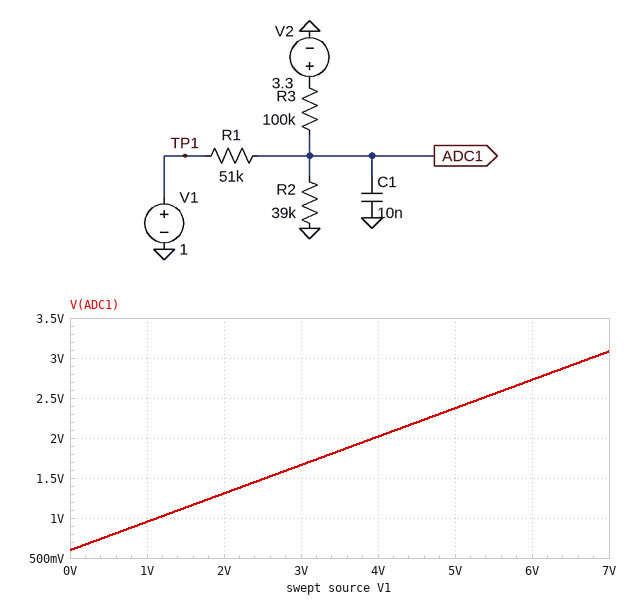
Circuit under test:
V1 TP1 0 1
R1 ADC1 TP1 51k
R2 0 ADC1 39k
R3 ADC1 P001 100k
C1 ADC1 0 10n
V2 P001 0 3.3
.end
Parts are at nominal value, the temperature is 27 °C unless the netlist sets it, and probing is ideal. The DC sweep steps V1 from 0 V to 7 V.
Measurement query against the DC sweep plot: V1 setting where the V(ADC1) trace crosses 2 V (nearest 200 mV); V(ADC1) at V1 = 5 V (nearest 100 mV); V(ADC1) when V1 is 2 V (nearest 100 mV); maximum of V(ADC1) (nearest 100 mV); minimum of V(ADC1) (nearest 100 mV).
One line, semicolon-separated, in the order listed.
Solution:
4.0 V; 2.4 V; 1.3 V; 3.1 V; 600 mV
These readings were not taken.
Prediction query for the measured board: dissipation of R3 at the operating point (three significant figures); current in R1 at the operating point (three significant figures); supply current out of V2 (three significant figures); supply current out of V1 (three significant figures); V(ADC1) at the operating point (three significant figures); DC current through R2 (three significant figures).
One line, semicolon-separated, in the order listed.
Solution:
55.1 µW; 937 nA; 23.5 µA; 937 nA; 952 mV; 24.4 µA
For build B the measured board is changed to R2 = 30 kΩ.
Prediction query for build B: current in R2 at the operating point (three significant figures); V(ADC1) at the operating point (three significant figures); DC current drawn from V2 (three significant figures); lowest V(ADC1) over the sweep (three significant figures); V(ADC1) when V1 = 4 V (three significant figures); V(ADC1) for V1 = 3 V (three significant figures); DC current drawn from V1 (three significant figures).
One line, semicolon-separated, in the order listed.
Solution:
27.9 µA; 836 mV; 24.6 µA; 524 mV; 1.77 V; 1.46 V; 3.22 µA
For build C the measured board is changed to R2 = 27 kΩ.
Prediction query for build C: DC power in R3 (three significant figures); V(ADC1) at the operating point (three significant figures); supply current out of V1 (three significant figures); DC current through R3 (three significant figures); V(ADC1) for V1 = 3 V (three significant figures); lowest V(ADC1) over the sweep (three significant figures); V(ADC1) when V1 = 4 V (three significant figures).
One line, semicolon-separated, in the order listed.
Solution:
63.0 µW; 789 mV; 4.13 µA; 25.1 µA; 1.38 V; 495 mV; 1.67 V
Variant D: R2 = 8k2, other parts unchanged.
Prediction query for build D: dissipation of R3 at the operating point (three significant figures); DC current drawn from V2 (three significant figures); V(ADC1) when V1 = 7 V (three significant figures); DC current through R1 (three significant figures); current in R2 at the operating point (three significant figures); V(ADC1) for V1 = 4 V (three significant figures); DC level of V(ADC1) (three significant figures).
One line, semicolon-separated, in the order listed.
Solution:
87.2 µW; 29.5 µA; 1.12 V; 12.8 µA; 42.3 µA; 735 mV; 347 mV
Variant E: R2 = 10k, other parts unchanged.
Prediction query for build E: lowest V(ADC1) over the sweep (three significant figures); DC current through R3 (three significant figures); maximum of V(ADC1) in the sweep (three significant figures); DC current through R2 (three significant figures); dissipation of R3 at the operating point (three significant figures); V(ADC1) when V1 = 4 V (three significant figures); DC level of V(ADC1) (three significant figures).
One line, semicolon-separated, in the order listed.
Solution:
255 mV; 28.9 µA; 1.31 V; 40.6 µA; 83.8 µW; 860 mV; 406 mV
